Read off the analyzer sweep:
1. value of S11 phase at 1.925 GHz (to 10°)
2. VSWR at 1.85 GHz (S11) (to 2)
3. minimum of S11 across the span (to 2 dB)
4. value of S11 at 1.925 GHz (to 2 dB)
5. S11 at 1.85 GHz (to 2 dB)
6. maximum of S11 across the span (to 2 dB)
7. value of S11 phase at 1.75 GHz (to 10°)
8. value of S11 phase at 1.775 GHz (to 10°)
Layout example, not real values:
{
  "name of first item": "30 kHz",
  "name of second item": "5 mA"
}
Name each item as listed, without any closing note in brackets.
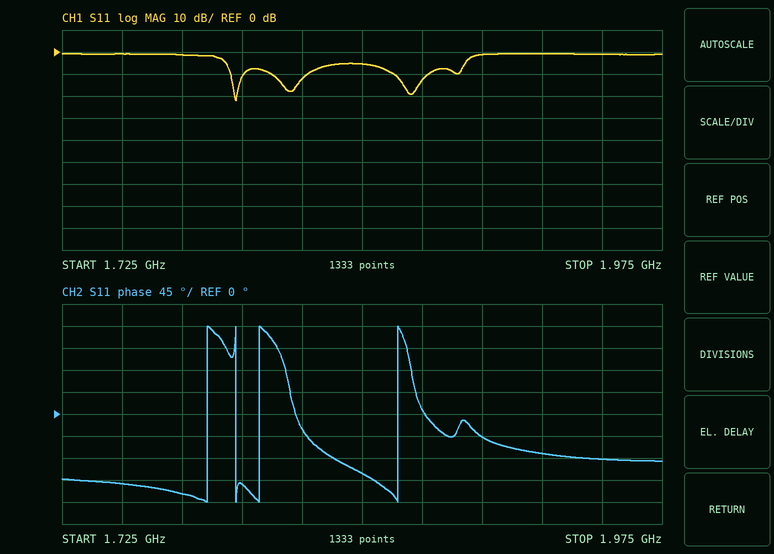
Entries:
{
  "value of S11 phase at 1.925 GHz": "-80°",
  "VSWR at 1.85 GHz (S11)": "4",
  "minimum of S11 across the span": "-22 dB",
  "value of S11 at 1.925 GHz": "0 dB",
  "S11 at 1.85 GHz": "-6 dB",
  "maximum of S11 across the span": "0 dB",
  "value of S11 phase at 1.75 GHz": "-140°",
  "value of S11 phase at 1.775 GHz": "-160°"
}
